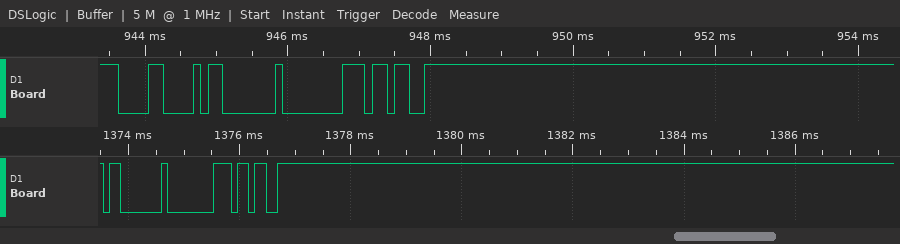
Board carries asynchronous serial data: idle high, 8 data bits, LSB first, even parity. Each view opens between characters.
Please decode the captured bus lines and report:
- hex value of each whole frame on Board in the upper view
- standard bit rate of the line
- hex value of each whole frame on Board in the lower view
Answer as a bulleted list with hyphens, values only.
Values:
- 18, 03, 80, 9B
- 9600 baud
- 03, 80, 9B
